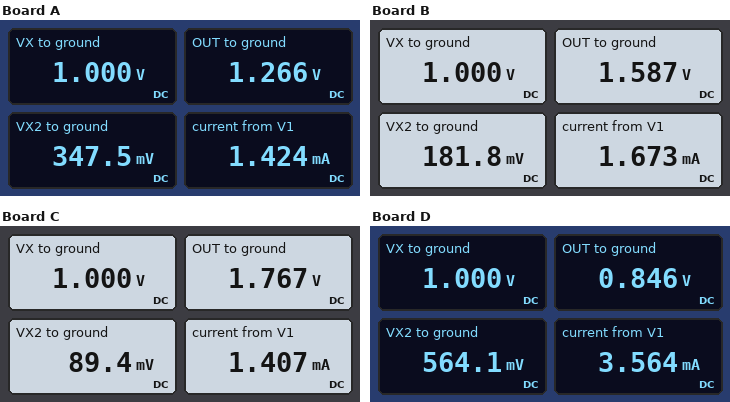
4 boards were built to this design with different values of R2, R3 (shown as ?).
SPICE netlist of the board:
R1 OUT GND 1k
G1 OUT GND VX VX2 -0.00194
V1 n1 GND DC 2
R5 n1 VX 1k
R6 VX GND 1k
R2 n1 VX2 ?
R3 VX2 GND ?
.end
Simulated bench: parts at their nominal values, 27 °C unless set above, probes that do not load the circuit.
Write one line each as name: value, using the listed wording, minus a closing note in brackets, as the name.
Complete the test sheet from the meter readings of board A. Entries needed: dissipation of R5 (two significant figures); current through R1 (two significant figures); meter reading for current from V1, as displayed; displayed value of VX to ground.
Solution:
dissipation of R5: 1.0 mW
current through R1: 1.3 mA
meter reading for current from V1, as displayed: 1.424 mA
displayed value of VX to ground: 1.000 V
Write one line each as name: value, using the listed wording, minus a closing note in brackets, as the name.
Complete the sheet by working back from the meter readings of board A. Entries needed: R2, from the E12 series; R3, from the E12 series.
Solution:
R2, from the E12 series: 3.9 kΩ
R3, from the E12 series: 820 Ω
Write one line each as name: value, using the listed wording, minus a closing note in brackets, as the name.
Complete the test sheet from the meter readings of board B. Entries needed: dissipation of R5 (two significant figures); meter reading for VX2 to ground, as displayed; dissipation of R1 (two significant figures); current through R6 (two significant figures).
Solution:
dissipation of R5: 1.0 mW
meter reading for VX2 to ground, as displayed: 181.8 mV
dissipation of R1: 2.5 mW
current through R6: 1.0 mA
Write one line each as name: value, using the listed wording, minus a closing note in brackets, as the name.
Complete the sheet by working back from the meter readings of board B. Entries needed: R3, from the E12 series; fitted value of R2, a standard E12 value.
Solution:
R3, from the E12 series: 270 Ω
fitted value of R2, a standard E12 value: 2.7 kΩ
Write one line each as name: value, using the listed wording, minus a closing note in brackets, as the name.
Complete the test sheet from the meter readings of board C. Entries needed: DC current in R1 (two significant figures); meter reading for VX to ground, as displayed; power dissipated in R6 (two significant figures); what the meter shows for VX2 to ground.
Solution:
DC current in R1: 1.8 mA
meter reading for VX to ground, as displayed: 1.000 V
power dissipated in R6: 1.0 mW
what the meter shows for VX2 to ground: 89.4 mV
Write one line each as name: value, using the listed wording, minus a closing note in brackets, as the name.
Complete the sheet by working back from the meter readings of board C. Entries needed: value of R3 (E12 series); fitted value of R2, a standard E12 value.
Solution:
value of R3: 220 Ω
fitted value of R2, a standard E12 value: 4.7 kΩ
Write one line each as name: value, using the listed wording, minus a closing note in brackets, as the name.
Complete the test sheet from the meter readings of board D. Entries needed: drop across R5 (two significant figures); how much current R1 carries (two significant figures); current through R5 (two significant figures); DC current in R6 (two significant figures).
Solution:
drop across R5: 1.0 V
how much current R1 carries: 850 µA
current through R5: 1.0 mA
DC current in R6: 1.0 mA
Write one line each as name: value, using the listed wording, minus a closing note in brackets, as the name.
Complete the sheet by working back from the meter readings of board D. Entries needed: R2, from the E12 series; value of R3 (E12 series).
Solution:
R2, from the E12 series: 560 Ω
value of R3: 220 Ω
